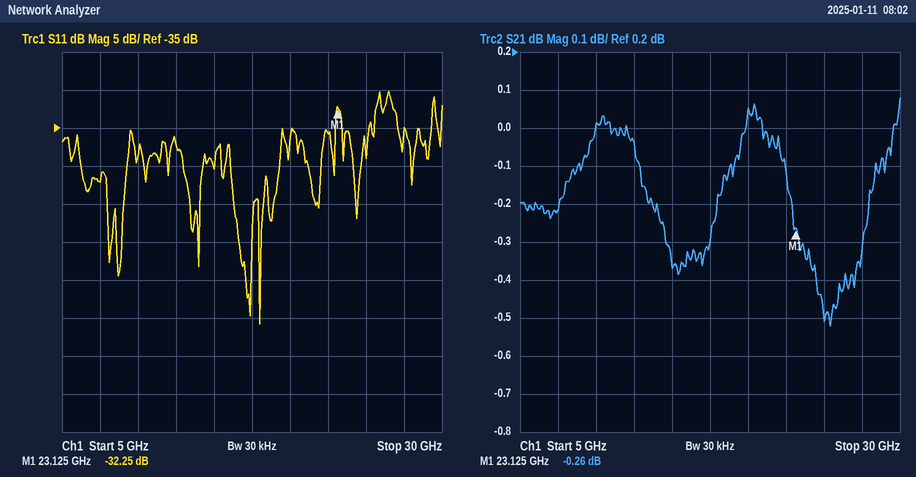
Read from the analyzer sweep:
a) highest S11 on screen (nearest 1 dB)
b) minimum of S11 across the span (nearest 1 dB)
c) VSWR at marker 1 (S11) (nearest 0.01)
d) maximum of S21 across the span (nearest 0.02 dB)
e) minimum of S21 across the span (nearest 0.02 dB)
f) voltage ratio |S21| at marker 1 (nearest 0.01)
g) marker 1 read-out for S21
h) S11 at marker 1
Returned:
-30 dB
-61 dB
1.05
0.08 dB
-0.52 dB
0.97
-0.26 dB
-32.25 dB
